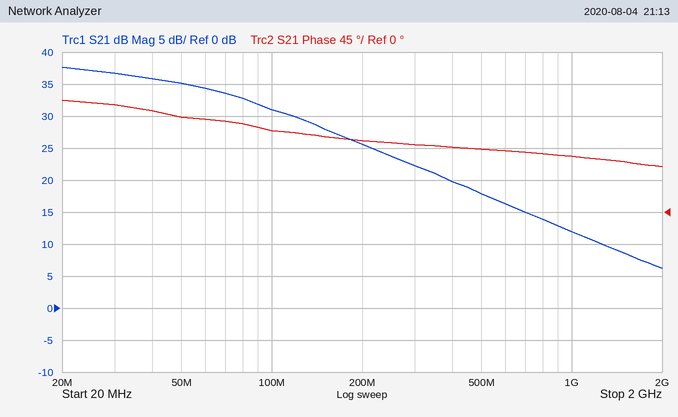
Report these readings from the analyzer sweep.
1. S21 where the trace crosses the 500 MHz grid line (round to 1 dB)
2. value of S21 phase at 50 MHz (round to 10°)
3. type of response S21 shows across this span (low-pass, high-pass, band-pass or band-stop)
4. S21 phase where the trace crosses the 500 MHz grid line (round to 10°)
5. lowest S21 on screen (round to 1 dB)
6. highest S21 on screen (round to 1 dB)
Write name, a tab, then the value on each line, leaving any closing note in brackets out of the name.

S21 where the trace crosses the 500 MHz grid line	18 dB
value of S21 phase at 50 MHz	130°
type of response S21 shows across this span	low-pass
S21 phase where the trace crosses the 500 MHz grid line	90°
lowest S21 on screen	6 dB
highest S21 on screen	38 dB
